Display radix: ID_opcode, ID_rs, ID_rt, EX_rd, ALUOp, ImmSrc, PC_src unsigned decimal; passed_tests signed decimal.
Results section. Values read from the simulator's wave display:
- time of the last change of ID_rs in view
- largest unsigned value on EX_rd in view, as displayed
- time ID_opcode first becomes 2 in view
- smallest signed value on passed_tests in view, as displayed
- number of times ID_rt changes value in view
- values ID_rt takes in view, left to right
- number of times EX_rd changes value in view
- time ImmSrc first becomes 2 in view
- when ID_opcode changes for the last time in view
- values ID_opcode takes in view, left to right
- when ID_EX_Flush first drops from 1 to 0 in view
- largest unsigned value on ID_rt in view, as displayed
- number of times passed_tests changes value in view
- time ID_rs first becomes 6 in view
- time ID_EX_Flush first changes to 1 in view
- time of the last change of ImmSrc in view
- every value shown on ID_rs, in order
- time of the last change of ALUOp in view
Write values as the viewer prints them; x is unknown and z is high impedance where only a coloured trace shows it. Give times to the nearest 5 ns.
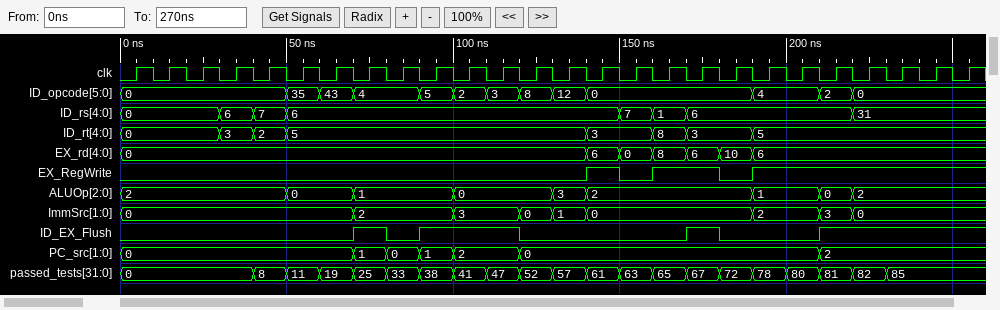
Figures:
220 ns
10
100 ns
0
7
0, 3, 2, 5, 3, 8, 3, 5
6
70 ns
220 ns
0, 35, 43, 4, 5, 2, 3, 8, 12, 0, 4, 2, 0
80 ns
8
20
30 ns
70 ns
220 ns
0, 6, 7, 6, 7, 1, 6, 31
220 ns
